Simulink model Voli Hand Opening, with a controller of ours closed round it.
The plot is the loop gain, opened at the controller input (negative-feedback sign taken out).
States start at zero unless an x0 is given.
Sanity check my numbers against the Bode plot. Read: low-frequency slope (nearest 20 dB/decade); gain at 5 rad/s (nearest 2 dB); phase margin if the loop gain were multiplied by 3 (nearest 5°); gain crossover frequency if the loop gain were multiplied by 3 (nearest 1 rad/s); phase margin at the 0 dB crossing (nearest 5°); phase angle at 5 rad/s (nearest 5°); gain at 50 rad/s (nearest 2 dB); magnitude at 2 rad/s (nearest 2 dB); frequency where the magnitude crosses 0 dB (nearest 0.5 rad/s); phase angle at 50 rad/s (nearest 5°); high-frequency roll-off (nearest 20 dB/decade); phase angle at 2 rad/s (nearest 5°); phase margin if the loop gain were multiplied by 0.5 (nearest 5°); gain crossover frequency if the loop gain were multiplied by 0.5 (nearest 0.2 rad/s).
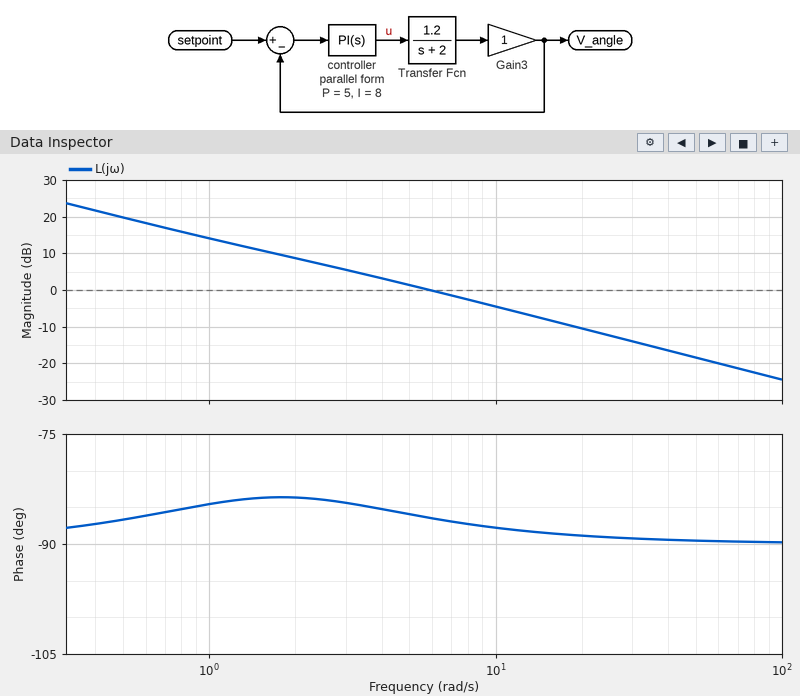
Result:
-20 dB/decade
2 dB
90°
18 rad/s
95°
-85°
-18 dB
8 dB
6.0 rad/s
-90°
-20 dB/decade
-85°
95°
2.8 rad/s
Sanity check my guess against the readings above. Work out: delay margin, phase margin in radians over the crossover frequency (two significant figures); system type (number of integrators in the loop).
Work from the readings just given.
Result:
0.28 s
1
